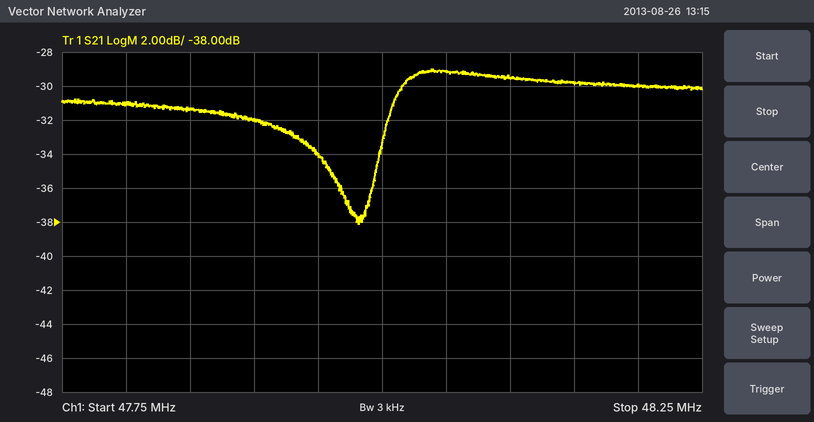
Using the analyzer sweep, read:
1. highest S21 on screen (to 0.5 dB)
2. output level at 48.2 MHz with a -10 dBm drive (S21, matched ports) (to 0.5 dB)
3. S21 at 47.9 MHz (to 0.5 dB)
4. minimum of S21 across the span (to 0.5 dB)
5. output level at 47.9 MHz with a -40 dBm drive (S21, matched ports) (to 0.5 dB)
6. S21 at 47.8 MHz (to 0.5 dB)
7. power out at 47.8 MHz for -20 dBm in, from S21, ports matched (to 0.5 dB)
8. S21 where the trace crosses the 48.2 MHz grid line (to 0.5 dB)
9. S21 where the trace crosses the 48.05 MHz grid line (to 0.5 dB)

-29.0 dB
-40.0 dBm
-32.0 dB
-38.0 dB
-72.0 dBm
-31.0 dB
-51.0 dBm
-30.0 dB
-29.0 dB
